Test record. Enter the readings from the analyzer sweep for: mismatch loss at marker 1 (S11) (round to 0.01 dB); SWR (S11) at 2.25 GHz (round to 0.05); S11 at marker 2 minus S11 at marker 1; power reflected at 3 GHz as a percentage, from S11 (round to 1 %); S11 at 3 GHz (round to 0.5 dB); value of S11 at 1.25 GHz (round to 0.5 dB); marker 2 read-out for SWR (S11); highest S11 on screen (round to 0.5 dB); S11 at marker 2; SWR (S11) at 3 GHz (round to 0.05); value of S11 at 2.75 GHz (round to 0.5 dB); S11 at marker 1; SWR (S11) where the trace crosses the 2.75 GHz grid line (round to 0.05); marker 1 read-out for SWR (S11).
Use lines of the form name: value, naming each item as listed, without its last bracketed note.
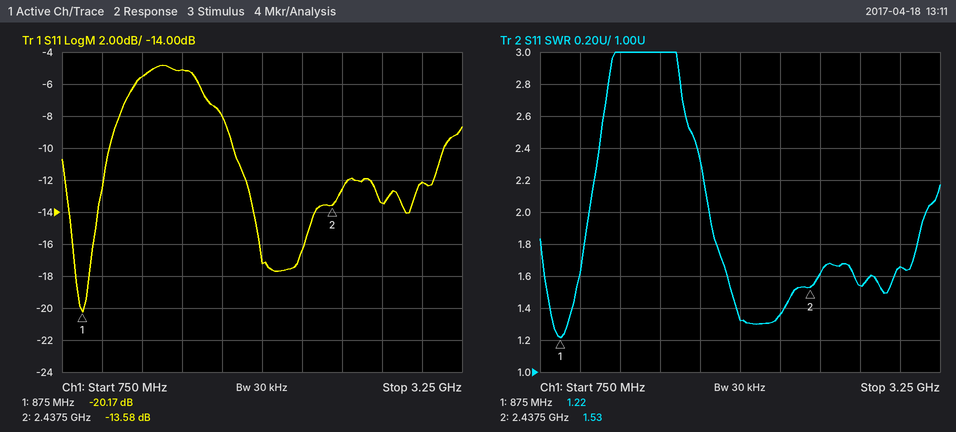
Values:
mismatch loss at marker 1 (S11): 0.04 dB
SWR (S11) at 2.25 GHz: 1.35
S11 at marker 2 minus S11 at marker 1: 6.59 dB
power reflected at 3 GHz as a percentage, from S11: 6 %
S11 at 3 GHz: -12.0 dB
value of S11 at 1.25 GHz: -5.5 dB
marker 2 read-out for SWR: 1.53
highest S11 on screen: -5.0 dB
S11 at marker 2: -13.58 dB
SWR (S11) at 3 GHz: 1.65
value of S11 at 2.75 GHz: -13.5 dB
S11 at marker 1: -20.17 dB
SWR (S11) where the trace crosses the 2.75 GHz grid line: 1.55
marker 1 read-out for SWR: 1.22
